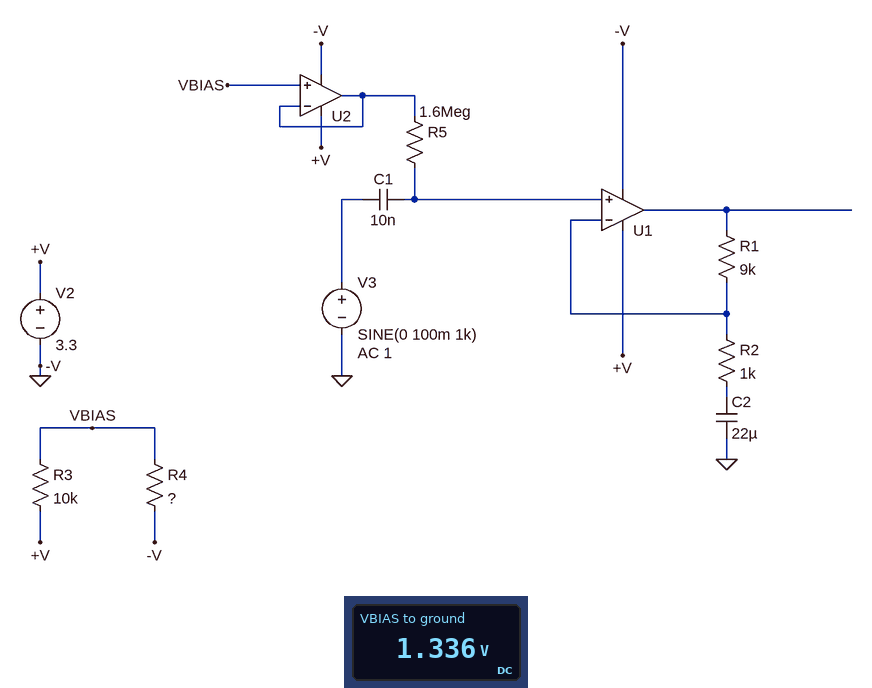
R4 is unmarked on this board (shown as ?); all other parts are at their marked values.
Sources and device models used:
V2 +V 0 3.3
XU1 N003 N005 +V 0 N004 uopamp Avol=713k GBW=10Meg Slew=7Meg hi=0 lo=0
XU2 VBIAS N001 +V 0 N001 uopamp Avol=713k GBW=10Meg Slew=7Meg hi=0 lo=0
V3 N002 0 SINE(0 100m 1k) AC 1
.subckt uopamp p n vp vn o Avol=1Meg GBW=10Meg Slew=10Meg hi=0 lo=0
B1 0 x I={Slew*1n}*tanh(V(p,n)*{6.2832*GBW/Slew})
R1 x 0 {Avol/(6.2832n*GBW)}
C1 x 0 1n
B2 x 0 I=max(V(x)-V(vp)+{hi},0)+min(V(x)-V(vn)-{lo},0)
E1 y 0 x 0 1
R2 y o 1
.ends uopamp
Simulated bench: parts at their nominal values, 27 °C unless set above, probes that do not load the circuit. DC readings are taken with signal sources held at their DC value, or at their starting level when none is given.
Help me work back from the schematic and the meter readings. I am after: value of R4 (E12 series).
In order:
6.8 kΩ
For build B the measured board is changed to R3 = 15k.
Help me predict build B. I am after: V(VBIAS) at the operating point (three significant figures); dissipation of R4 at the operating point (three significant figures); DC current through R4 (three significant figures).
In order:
1.03 V
156 µW
151 µA
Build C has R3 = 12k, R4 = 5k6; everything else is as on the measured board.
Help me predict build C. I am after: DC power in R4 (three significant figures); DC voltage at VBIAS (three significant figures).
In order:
197 µW
1.05 V
